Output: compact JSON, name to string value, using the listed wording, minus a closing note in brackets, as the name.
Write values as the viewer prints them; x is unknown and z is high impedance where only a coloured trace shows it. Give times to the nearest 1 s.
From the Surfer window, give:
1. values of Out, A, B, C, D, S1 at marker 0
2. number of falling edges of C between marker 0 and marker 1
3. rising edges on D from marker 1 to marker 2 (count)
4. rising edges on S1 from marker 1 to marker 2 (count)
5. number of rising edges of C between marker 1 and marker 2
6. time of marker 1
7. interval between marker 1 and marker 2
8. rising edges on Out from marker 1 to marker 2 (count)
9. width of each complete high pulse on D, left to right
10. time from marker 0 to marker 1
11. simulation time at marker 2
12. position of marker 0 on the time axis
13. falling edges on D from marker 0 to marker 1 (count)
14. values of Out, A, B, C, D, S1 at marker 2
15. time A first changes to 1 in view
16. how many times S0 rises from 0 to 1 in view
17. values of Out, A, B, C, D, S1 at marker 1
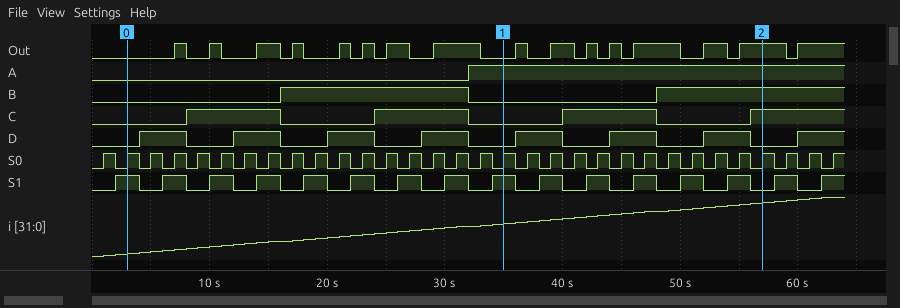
{"values of Out, A, B, C, D, S1 at marker 0": "Out=0, A=0, B=0, C=0, D=0, S1=1", "number of falling edges of C between marker 0 and marker 1": "2", "rising edges on D from marker 1 to marker 2": "3", "rising edges on S1 from marker 1 to marker 2": "5", "number of rising edges of C between marker 1 and marker 2": "2", "time of marker 1": "35 s", "interval between marker 1 and marker 2": "22 s", "rising edges on Out from marker 1 to marker 2": "7", "width of each complete high pulse on D, left to right": "4 s, 4 s, 4 s, 4 s, 4 s, 4 s, 4 s", "time from marker 0 to marker 1": "32 s", "simulation time at marker 2": "57 s", "position of marker 0 on the time axis": "3 s", "falling edges on D from marker 0 to marker 1": "4", "values of Out, A, B, C, D, S1 at marker 2": "Out=1, A=1, B=1, C=1, D=0, S1=0", "time A first changes to 1 in view": "32 s", "how many times S0 rises from 0 to 1 in view": "32", "values of Out, A, B, C, D, S1 at marker 1": "Out=0, A=1, B=0, C=0, D=0, S1=1"}
